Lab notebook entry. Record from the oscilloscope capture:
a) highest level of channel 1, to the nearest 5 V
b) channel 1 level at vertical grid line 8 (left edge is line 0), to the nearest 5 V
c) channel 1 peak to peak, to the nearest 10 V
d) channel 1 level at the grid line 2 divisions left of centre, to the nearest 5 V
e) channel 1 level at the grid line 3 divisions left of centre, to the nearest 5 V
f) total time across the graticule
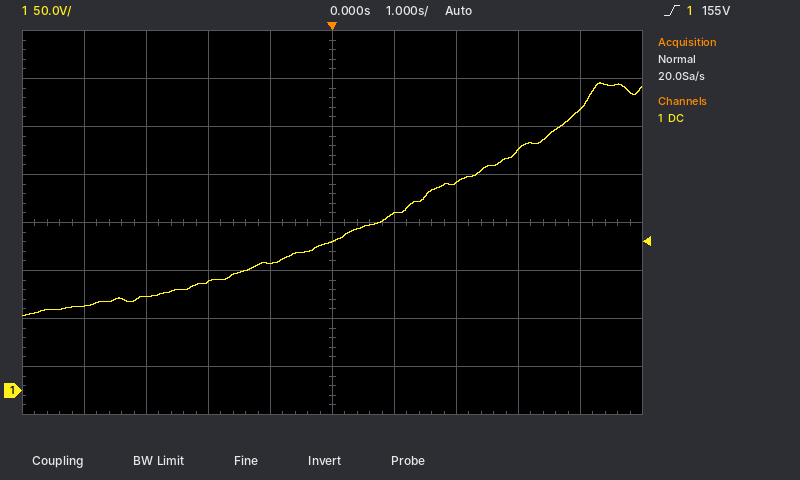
320 V
250 V
240 V
115 V
100 V
10 s
